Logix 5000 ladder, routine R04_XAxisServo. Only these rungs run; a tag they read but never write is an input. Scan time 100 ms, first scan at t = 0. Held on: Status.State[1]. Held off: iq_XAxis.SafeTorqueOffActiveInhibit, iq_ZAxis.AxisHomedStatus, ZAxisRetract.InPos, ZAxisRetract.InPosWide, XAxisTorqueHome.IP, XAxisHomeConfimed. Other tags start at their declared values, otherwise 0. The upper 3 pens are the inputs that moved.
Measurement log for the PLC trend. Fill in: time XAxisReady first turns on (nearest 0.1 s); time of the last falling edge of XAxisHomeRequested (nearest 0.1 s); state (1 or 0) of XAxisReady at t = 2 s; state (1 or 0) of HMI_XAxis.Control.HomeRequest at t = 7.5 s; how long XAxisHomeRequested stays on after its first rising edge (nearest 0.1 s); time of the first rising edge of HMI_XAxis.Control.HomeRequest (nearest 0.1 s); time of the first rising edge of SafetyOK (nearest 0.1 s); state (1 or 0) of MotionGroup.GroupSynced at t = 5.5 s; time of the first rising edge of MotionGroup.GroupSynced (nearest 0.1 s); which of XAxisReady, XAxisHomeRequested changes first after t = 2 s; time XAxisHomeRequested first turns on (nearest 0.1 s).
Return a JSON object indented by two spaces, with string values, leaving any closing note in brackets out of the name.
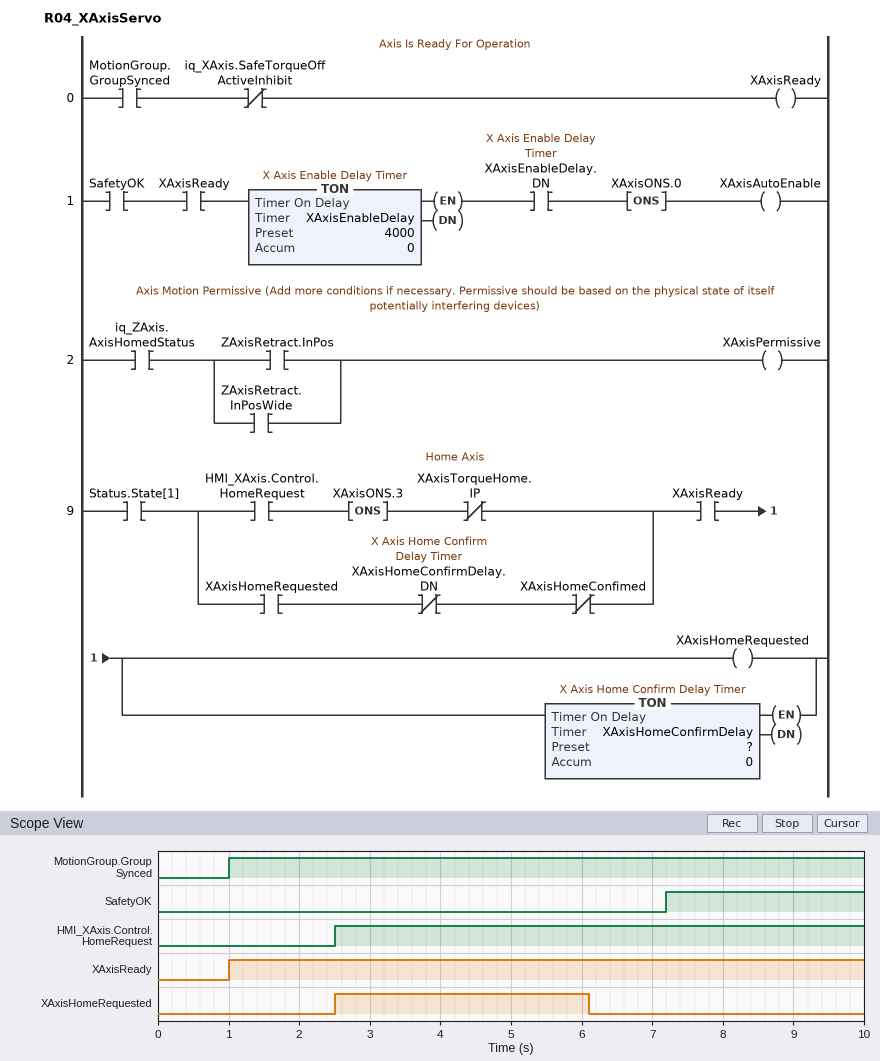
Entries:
{
  "time XAxisReady first turns on": "1.0 s",
  "time of the last falling edge of XAxisHomeRequested": "6.1 s",
  "state (1 or 0) of XAxisReady at t = 2 s": "1",
  "state (1 or 0) of HMI_XAxis.Control.HomeRequest at t = 7.5 s": "1",
  "how long XAxisHomeRequested stays on after its first rising edge": "3.6 s",
  "time of the first rising edge of HMI_XAxis.Control.HomeRequest": "2.5 s",
  "time of the first rising edge of SafetyOK": "7.2 s",
  "state (1 or 0) of MotionGroup.GroupSynced at t = 5.5 s": "1",
  "time of the first rising edge of MotionGroup.GroupSynced": "1.0 s",
  "which of XAxisReady, XAxisHomeRequested changes first after t = 2 s": "XAxisHomeRequested",
  "time XAxisHomeRequested first turns on": "2.5 s"
}
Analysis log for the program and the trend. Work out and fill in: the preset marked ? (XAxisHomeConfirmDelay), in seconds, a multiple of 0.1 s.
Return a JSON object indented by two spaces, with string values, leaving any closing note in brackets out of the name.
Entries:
{
  "the preset marked ? (XAxisHomeConfirmDelay), in seconds, a multiple of 0.1 s": "3.5 s"
}
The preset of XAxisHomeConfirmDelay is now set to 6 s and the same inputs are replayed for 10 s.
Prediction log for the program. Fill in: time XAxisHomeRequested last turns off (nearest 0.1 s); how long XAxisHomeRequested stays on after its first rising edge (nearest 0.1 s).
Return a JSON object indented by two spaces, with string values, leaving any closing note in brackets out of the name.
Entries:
{
  "time XAxisHomeRequested last turns off": "8.6 s",
  "how long XAxisHomeRequested stays on after its first rising edge": "6.1 s"
}
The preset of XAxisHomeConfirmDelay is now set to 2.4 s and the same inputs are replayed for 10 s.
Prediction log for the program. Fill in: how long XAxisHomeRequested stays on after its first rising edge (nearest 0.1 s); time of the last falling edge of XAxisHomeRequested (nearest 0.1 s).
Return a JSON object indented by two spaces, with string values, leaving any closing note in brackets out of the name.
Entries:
{
  "how long XAxisHomeRequested stays on after its first rising edge": "2.5 s",
  "time of the last falling edge of XAxisHomeRequested": "5.0 s"
}
